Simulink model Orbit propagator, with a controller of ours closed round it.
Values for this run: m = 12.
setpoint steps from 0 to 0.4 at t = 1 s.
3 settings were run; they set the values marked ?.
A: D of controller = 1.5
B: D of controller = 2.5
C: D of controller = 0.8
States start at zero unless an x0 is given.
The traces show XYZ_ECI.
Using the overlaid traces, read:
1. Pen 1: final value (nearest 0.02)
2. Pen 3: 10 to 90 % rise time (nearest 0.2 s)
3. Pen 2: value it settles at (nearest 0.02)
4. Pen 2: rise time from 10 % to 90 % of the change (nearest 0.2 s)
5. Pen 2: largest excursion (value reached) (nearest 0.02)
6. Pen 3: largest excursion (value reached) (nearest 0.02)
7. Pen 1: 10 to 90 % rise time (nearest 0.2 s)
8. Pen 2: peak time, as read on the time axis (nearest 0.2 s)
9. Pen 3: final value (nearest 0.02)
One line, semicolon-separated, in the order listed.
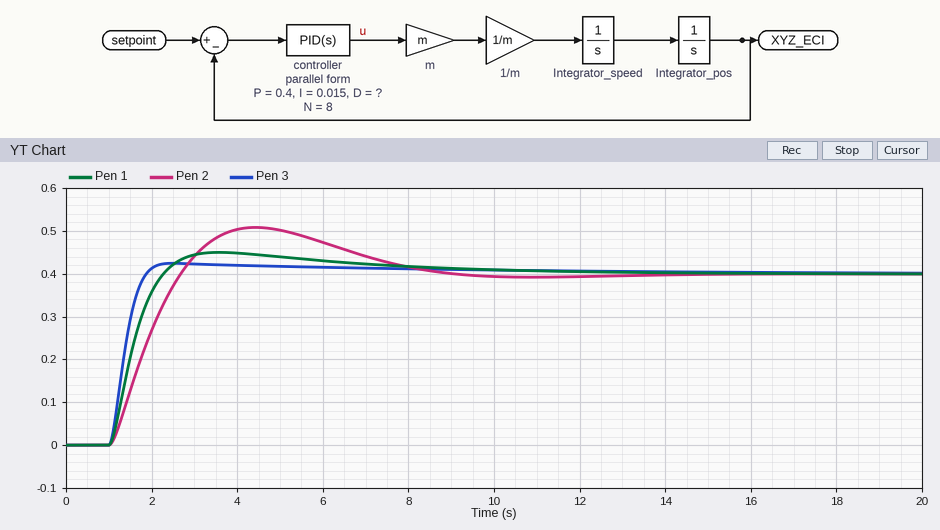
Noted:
0.40; 0.6 s; 0.40; 1.2 s; 0.50; 0.42; 0.8 s; 4.4 s; 0.40
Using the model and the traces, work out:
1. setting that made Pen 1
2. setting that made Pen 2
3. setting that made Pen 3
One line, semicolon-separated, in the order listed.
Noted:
A; C; B
